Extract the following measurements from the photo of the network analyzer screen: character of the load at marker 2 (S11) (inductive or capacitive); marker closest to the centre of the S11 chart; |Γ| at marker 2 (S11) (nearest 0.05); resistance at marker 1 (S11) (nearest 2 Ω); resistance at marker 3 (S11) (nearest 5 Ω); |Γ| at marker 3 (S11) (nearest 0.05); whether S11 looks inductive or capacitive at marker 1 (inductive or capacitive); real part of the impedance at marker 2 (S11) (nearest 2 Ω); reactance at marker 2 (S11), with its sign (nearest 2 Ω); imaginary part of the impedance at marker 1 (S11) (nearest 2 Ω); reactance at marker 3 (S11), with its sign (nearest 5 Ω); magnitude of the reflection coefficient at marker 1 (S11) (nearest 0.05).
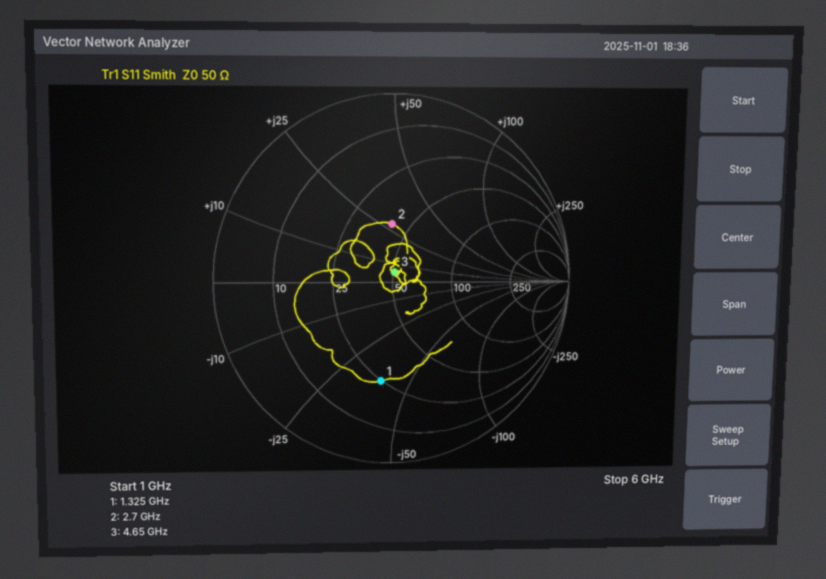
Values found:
inductive
marker 3
0.30
24 Ω
50 Ω
0.05
capacitive
40 Ω
+28 Ω
-38 Ω
+5 Ω
0.55
